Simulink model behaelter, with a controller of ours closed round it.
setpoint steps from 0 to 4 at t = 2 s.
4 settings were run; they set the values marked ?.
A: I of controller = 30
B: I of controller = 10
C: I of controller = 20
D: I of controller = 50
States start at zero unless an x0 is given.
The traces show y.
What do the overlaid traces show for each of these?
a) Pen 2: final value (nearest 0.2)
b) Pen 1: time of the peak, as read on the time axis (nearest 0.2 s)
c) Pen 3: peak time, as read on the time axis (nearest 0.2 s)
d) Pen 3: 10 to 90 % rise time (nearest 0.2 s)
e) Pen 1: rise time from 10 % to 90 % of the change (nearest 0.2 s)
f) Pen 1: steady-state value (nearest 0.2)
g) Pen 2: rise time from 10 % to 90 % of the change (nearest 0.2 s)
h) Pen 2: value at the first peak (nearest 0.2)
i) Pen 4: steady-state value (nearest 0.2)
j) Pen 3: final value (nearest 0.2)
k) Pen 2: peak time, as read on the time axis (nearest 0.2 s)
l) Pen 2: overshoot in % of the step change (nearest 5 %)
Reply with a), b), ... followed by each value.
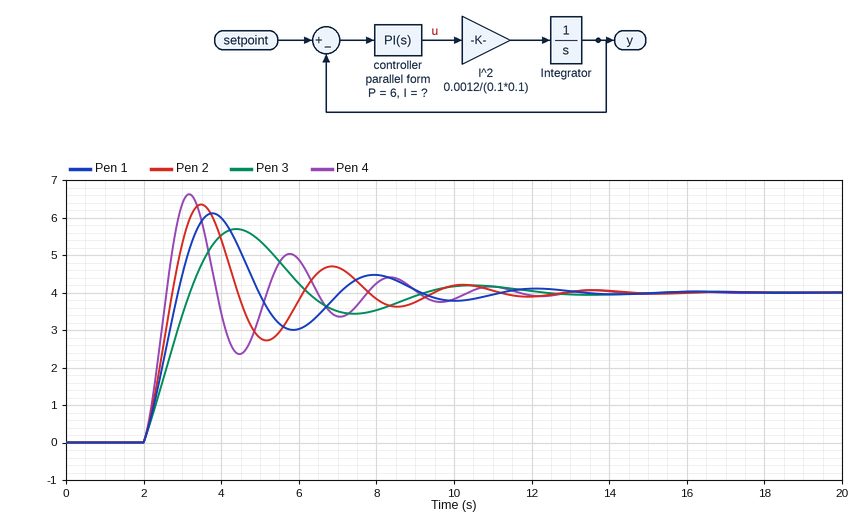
a) 4.0
b) 3.8 s
c) 4.4 s
d) 1.0 s
e) 0.6 s
f) 4.0
g) 0.6 s
h) 6.4
i) 4.0
j) 4.0
k) 3.4 s
l) 60 %
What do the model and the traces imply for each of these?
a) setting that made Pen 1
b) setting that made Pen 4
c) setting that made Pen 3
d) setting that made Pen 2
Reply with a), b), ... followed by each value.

a) C
b) D
c) B
d) A
